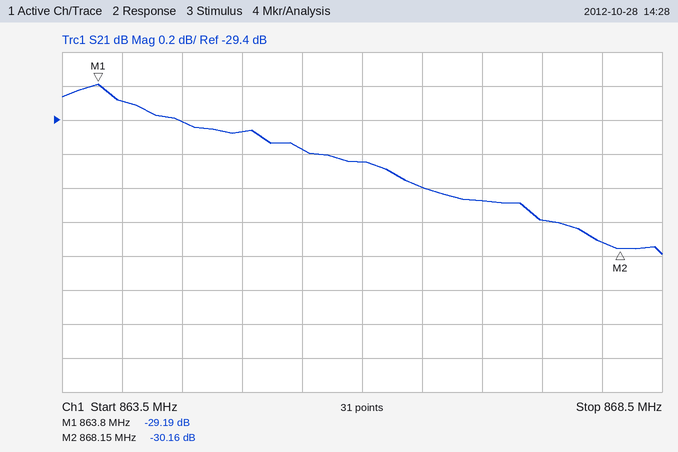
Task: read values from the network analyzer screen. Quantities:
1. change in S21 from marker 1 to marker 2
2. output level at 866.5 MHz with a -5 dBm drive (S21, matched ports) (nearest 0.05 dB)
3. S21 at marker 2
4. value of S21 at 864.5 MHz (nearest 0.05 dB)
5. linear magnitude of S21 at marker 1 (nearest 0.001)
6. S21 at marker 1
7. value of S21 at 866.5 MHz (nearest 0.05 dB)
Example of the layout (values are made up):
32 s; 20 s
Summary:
-0.97 dB; -34.80 dBm; -30.16 dB; -29.40 dB; 0.035; -29.19 dB; -29.80 dB
